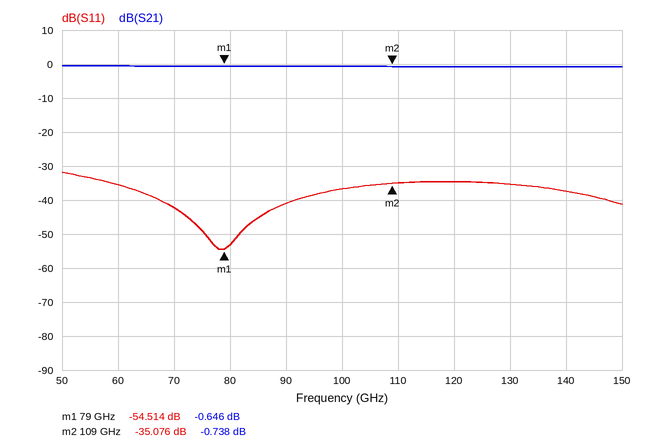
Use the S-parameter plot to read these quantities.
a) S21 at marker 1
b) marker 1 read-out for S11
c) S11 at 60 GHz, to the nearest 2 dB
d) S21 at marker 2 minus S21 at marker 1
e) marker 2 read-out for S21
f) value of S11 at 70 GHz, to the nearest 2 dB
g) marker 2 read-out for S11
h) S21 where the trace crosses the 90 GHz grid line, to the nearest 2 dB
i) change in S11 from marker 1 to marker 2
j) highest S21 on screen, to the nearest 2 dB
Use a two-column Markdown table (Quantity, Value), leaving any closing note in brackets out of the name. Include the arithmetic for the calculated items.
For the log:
| Quantity | Value |
|---|---|
| S21 at marker 1 | -0.646 dB |
| marker 1 read-out for S11 | -54.514 dB |
| S11 at 60 GHz, to the nearest 2 dB | -36 dB |
| S21 at marker 2 minus S21 at marker 1 | -0.738 − (-0.646) = -0.092 dB |
| marker 2 read-out for S21 | -0.738 dB |
| value of S11 at 70 GHz, to the nearest 2 dB | -42 dB |
| marker 2 read-out for S11 | -35.076 dB |
| S21 where the trace crosses the 90 GHz grid line, to the nearest 2 dB | 0 dB |
| change in S11 from marker 1 to marker 2 | -35.076 − (-54.514) = 19.438 dB |
| highest S21 on screen, to the nearest 2 dB | 0 dB |
